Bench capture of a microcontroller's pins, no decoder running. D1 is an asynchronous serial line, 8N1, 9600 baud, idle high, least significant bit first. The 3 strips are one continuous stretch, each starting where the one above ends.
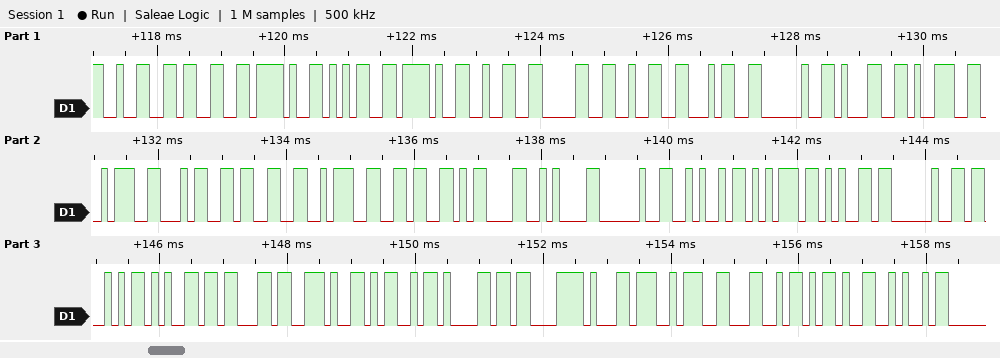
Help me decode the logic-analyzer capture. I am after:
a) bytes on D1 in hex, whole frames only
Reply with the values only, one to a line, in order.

32 33 2F 35 2F 32 30 32 34 20 31 39 3A 34 33 3A 36 0D 0A 20 4A 75 65 20 53 65 63 2E 4D 61 C3 B1 3A 4C 2D 4A
